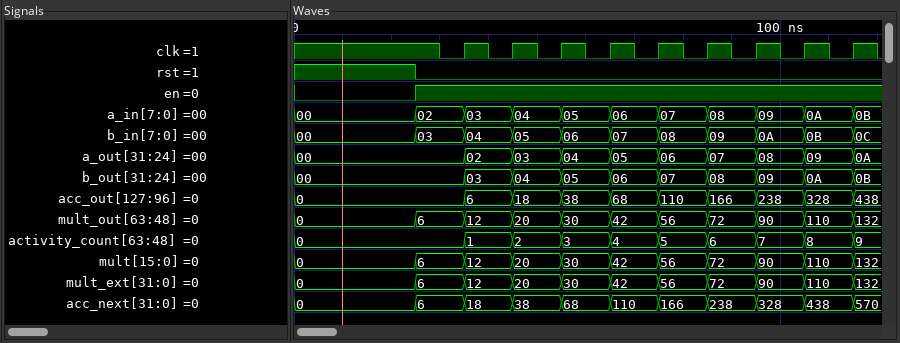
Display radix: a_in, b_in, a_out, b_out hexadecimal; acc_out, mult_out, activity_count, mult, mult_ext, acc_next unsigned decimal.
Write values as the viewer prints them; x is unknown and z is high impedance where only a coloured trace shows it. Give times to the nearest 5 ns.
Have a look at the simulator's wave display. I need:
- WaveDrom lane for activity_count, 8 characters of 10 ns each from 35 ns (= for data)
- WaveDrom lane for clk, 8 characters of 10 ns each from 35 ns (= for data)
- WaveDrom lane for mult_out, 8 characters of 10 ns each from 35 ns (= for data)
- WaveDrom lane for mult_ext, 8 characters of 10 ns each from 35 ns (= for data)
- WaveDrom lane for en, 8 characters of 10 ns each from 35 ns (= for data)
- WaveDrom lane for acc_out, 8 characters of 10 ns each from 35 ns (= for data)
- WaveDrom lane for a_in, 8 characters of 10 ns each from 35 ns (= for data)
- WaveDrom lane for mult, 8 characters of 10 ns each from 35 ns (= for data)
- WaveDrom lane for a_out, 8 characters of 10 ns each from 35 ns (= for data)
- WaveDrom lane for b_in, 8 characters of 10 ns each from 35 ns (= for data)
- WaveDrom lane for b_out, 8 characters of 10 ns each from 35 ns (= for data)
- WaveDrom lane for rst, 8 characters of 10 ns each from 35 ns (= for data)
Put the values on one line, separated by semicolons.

{name: 'activity_count', wave: '========', data: '1 2 3 4 5 6 7 8'}; {name: 'clk', wave: 'p.......'}; {name: 'mult_out', wave: '========', data: '12 20 30 42 56 72 90 110'}; {name: 'mult_ext', wave: '========', data: '12 20 30 42 56 72 90 110'}; {name: 'en', wave: '1.......'}; {name: 'acc_out', wave: '========', data: '6 18 38 68 110 166 238 328'}; {name: 'a_in', wave: '========', data: '03 04 05 06 07 08 09 0A'}; {name: 'mult', wave: '========', data: '12 20 30 42 56 72 90 110'}; {name: 'a_out', wave: '========', data: '02 03 04 05 06 07 08 09'}; {name: 'b_in', wave: '========', data: '04 05 06 07 08 09 0A 0B'}; {name: 'b_out', wave: '========', data: '03 04 05 06 07 08 09 0A'}; {name: 'rst', wave: '0.......'}
